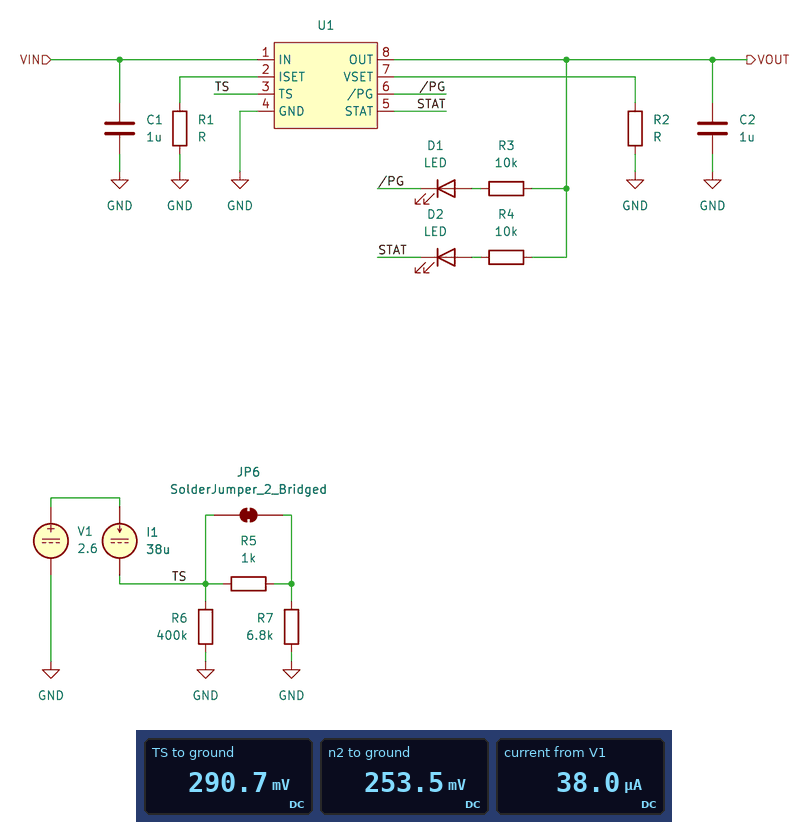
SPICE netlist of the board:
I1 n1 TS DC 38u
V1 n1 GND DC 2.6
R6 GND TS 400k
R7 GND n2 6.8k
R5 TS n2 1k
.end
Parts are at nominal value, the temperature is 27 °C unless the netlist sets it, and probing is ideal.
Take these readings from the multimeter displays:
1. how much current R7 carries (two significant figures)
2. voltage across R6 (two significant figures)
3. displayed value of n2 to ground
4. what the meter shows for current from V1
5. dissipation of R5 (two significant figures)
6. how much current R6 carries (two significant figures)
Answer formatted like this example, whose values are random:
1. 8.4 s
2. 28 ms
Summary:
1. 37 µA
2. 290 mV
3. 253.5 mV
4. 38.0 µA
5. 1.4 µW
6. 730 nA
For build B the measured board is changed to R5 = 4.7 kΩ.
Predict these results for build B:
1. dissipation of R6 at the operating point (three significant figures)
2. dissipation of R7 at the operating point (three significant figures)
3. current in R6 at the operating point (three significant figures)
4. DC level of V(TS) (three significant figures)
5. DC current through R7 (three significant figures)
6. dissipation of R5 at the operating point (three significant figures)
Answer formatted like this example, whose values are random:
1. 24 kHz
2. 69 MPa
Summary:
1. 451 nW
2. 9.28 µW
3. 1.06 µA
4. 425 mV
5. 36.9 µA
6. 6.41 µW
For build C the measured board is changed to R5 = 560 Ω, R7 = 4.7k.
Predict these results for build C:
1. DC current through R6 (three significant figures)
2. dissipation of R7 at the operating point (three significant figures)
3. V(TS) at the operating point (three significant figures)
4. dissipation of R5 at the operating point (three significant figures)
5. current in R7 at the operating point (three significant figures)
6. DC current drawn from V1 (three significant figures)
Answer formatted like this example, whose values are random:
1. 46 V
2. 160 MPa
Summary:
1. 493 nA
2. 6.61 µW
3. 197 mV
4. 788 nW
5. 37.5 µA
6. 38.0 µA
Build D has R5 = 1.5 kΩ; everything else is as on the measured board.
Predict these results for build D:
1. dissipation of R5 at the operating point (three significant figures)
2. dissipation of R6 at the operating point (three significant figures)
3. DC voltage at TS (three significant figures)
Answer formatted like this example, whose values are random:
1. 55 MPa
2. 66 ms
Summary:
1. 2.08 µW
2. 239 nW
3. 309 mV
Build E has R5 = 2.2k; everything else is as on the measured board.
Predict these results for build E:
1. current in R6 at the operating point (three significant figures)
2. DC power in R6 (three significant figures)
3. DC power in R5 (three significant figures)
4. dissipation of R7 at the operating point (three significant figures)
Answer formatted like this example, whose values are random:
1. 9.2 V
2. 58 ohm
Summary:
1. 836 nA
2. 280 nW
3. 3.04 µW
4. 9.39 µW
